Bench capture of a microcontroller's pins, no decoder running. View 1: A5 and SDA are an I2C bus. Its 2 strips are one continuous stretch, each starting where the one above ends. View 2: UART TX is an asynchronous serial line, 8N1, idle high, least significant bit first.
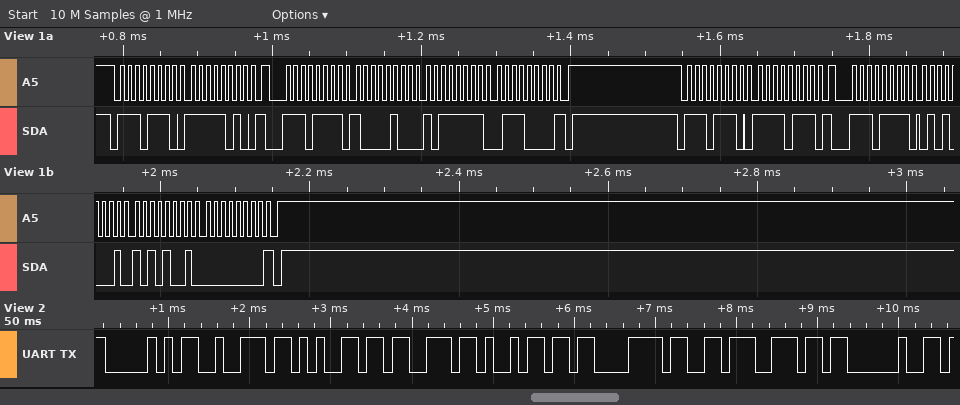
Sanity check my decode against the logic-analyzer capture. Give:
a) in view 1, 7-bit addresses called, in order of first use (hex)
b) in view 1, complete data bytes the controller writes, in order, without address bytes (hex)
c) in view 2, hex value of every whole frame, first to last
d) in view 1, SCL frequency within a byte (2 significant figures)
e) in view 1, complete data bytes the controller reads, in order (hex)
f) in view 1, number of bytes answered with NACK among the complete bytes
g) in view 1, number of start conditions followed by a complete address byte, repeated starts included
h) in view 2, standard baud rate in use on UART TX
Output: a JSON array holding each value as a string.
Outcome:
["0x77", "FA F7", "50 72 65 73 69 C3 B3 6E 20", "100 kHz", "84 BF 70 51 A9 00", "2", "4", "9600 baud"]
